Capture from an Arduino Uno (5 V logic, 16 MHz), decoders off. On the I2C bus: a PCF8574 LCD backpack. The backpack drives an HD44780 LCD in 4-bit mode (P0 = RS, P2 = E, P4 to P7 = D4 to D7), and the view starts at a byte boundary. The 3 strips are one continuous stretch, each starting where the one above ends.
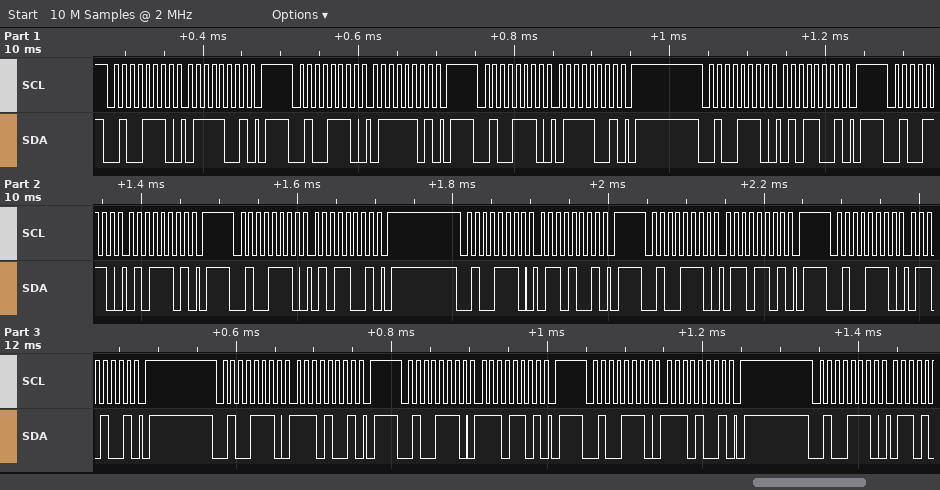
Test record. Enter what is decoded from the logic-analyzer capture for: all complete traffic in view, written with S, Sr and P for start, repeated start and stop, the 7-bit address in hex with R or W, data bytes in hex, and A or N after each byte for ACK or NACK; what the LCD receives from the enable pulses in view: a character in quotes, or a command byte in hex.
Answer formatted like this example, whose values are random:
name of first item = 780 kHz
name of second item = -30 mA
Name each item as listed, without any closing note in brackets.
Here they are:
all complete traffic in view, written with S, Sr and P for start, repeated start and stop, the 7-bit address in hex with R or W, data bytes in hex, and A or N after each byte for ACK or NACK = S 27W A 79 A P S 27W A 7D A P S 27W A 79 A P S 27W A 59 A P S 27W A 5D A P S 27W A 59 A P S 27W A 69 A P S 27W A 6D A P S 27W A 69 A P S 27W A E9 A P S 27W A ED A P S 27W A E9 A P S 27W A
what the LCD receives from the enable pulses in view: a character in quotes, or a command byte in hex = 'u' 'n'
